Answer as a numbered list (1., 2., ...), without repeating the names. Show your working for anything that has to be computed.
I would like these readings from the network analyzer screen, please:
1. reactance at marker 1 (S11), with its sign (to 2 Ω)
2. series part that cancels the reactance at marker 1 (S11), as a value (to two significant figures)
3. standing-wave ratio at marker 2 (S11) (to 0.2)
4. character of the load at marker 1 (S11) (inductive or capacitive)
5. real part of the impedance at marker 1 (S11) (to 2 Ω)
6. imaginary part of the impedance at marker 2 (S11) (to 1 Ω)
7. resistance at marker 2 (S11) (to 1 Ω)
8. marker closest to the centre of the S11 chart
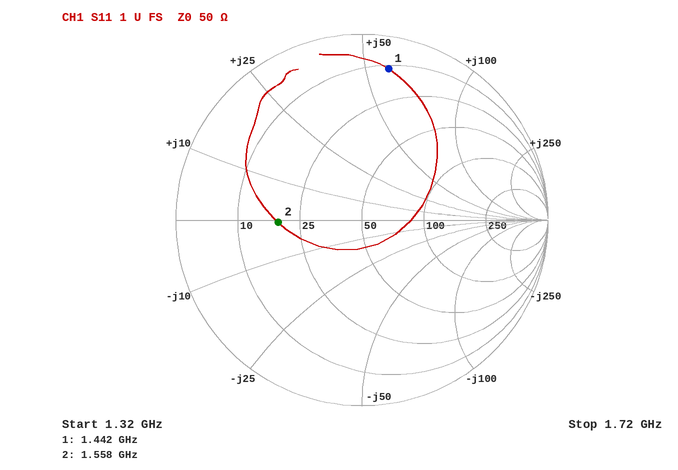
1. +58 Ω
2. C = 1/(2π × 1.442 GHz × 58 Ω) ≈ 1.9 pF
3. 2.6
4. inductive
5. 12 Ω
6. -1 Ω
7. 19 Ω
8. marker 2
